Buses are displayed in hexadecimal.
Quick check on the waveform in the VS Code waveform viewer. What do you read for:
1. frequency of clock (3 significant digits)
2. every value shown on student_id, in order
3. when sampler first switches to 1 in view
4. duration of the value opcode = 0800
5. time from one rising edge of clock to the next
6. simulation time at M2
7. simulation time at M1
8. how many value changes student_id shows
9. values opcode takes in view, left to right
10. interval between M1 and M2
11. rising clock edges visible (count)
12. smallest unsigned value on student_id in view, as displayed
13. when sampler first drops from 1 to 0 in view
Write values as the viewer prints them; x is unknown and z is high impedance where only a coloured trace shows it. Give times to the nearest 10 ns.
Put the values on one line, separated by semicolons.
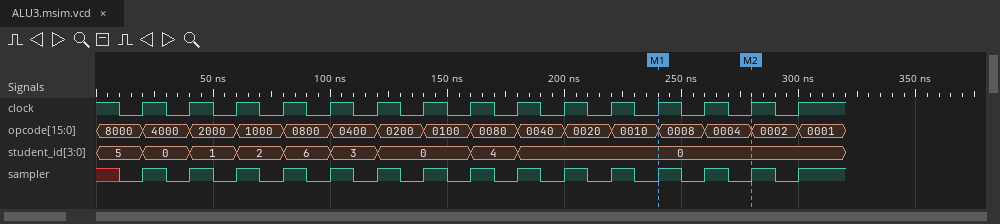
50.0 MHz; 5, 0, 1, 2, 6, 3, 0, 4, 0; 20 ns; 20 ns; 20 ns; 280 ns; 240 ns; 8; 8000, 4000, 2000, 1000, 0800, 0400, 0200, 0100, 0080, 0040, 0020, 0010, 0008, 0004, 0002, 0001; 40 ns; 15; 0; 30 ns
